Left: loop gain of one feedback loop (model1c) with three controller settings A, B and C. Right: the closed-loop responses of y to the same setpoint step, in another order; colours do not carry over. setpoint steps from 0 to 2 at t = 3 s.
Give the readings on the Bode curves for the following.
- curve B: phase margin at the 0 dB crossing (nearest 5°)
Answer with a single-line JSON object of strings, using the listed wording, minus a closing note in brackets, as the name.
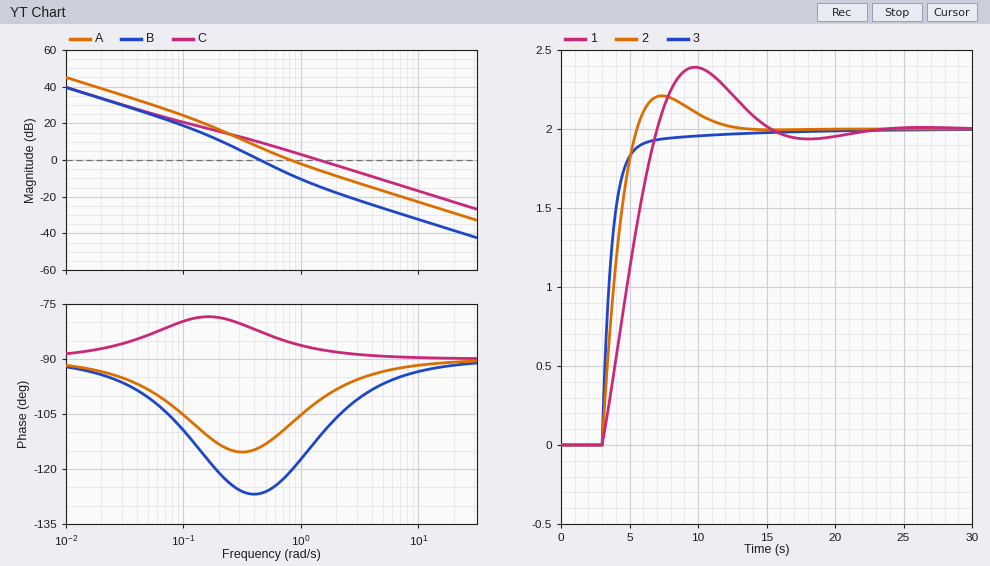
{"curve B: phase margin at the 0 dB crossing": "55°"}
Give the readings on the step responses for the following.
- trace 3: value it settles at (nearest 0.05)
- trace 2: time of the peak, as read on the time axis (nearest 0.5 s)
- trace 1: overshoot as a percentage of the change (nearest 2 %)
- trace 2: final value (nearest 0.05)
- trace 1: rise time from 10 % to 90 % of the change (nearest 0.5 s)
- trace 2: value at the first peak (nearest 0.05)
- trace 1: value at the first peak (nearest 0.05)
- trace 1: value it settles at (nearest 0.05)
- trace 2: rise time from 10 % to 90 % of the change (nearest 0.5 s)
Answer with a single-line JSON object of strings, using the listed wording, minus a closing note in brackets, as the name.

{"trace 3: value it settles at": "2.00", "trace 2: time of the peak, as read on the time axis": "7.5 s", "trace 1: overshoot as a percentage of the change": "20 %", "trace 2: final value": "2.00", "trace 1: rise time from 10 % to 90 % of the change": "3.0 s", "trace 2: value at the first peak": "2.20", "trace 1: value at the first peak": "2.40", "trace 1: value it settles at": "2.00", "trace 2: rise time from 10 % to 90 % of the change": "2.0 s"}
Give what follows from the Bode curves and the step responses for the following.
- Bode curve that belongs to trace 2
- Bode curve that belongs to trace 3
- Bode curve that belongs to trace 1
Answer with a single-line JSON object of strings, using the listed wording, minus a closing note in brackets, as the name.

{"Bode curve that belongs to trace 2": "A", "Bode curve that belongs to trace 3": "C", "Bode curve that belongs to trace 1": "B"}
